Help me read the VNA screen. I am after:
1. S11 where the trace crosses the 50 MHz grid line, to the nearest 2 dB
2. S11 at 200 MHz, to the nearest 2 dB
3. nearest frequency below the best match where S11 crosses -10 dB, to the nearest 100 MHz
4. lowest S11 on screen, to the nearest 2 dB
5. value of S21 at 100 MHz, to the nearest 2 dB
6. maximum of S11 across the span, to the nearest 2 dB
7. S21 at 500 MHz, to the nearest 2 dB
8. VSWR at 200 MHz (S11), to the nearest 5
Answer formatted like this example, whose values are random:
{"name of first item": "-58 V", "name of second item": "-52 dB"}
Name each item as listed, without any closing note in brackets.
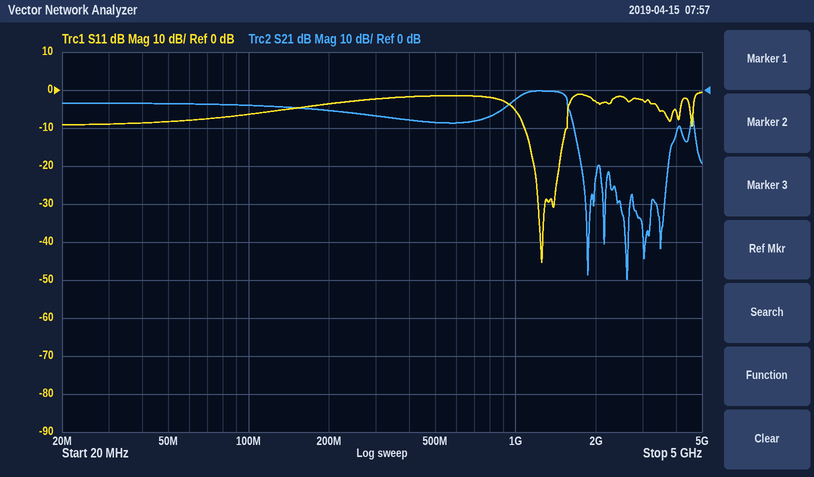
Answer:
{"S11 where the trace crosses the 50 MHz grid line, to the nearest 2 dB": "-8 dB", "S11 at 200 MHz, to the nearest 2 dB": "-4 dB", "nearest frequency below the best match where S11 crosses -10 dB, to the nearest 100 MHz": "1.1 GHz", "lowest S11 on screen, to the nearest 2 dB": "-46 dB", "value of S21 at 100 MHz, to the nearest 2 dB": "-4 dB", "maximum of S11 across the span, to the nearest 2 dB": "0 dB", "S21 at 500 MHz, to the nearest 2 dB": "-8 dB", "VSWR at 200 MHz (S11), to the nearest 5": "5"}
